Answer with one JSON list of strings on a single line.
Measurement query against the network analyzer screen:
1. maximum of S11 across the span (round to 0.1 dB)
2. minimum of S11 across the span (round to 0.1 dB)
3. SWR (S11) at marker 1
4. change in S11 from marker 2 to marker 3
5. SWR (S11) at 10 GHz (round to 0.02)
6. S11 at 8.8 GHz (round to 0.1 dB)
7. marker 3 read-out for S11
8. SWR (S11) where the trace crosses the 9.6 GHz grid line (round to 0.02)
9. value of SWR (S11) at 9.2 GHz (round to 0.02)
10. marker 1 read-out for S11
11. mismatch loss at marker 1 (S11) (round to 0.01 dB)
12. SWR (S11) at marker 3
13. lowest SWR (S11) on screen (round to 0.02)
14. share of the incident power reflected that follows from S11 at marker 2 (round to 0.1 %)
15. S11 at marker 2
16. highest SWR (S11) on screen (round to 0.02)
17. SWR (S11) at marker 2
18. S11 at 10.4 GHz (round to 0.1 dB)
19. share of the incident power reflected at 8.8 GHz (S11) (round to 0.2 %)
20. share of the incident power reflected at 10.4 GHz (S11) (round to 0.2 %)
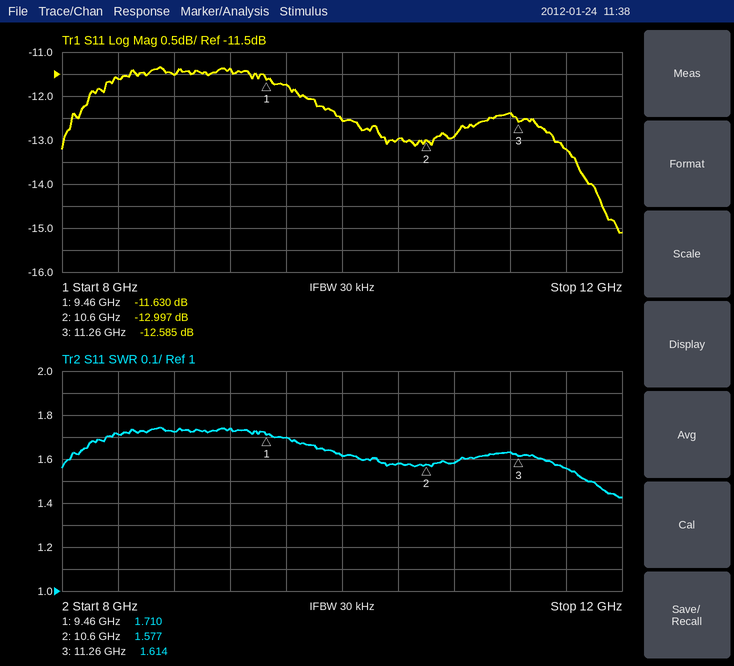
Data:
["-11.3 dB", "-15.1 dB", "1.710", "0.412 dB", "1.62", "-11.5 dB", "-12.585 dB", "1.70", "1.74", "-11.630 dB", "0.31 dB", "1.614", "1.42", "5.0 %", "-12.997 dB", "1.74", "1.577", "-13.0 dB", "7.0 %", "5.0 %"]
